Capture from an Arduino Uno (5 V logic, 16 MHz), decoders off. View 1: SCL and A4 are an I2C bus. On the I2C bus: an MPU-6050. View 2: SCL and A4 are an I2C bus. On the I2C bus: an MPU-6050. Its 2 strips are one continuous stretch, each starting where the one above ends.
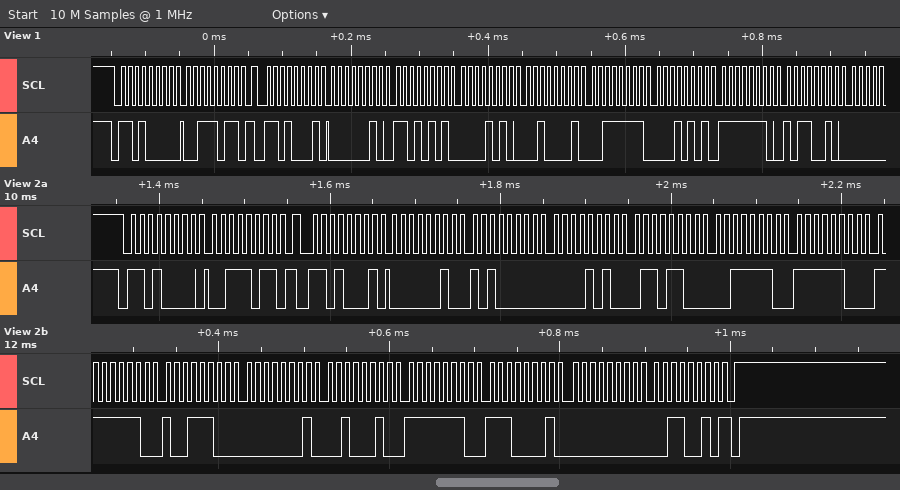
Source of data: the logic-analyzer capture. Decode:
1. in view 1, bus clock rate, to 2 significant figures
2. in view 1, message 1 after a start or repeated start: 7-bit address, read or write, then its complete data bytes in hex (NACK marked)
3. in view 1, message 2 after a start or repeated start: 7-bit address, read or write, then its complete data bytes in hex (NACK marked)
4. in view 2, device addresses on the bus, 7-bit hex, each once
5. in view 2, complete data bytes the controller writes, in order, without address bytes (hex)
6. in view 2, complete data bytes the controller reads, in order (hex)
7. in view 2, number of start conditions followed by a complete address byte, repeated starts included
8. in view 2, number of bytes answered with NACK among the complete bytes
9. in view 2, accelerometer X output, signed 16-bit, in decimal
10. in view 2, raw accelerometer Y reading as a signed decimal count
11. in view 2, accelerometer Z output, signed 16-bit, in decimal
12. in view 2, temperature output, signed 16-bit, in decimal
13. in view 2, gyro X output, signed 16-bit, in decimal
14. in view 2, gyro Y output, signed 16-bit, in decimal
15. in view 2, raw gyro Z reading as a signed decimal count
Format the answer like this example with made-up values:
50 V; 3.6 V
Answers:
100 kHz; 0x68 write: 3B; 0x68 read: 02 D5 0A 21 3F 15 FE B2; 0x68; 3B; 02 A0 0A 6C 3E FC FE 9C 01 22 FE E1 00 32; 2; 1; 672; 2668; 16124; -356; 290; -287; 50
